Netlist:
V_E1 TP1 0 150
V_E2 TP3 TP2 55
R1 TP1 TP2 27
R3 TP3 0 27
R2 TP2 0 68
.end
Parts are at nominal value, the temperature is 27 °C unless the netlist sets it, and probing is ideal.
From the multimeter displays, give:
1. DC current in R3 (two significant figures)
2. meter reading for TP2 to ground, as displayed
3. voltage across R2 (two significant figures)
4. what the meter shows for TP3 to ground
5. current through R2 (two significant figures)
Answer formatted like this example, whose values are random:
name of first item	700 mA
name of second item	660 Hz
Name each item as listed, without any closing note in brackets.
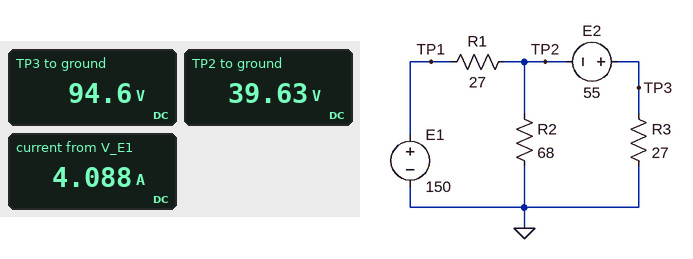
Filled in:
DC current in R3	3.5 A
meter reading for TP2 to ground, as displayed	39.63 V
voltage across R2	40 V
what the meter shows for TP3 to ground	94.6 V
current through R2	580 mA
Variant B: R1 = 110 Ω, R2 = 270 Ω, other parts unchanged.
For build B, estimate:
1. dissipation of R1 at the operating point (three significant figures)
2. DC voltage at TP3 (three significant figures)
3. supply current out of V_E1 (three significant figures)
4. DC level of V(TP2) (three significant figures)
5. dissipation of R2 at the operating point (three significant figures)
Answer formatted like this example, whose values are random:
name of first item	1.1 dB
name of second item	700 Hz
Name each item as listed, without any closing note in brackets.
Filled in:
dissipation of R1 at the operating point	243 W
DC voltage at TP3	41.5 V
supply current out of V_E1	1.49 A
DC level of V(TP2)	-13.5 V
dissipation of R2 at the operating point	676 mW
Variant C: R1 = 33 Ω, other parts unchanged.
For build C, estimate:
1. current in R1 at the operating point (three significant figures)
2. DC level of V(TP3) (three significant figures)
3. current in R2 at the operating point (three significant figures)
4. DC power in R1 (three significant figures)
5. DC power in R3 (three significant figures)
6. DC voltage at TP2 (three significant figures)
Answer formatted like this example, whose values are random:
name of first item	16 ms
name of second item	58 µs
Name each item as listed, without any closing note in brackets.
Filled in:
current in R1 at the operating point	3.62 A
DC level of V(TP3)	85.6 V
current in R2 at the operating point	450 mA
DC power in R1	432 W
DC power in R3	271 W
DC voltage at TP2	30.6 V
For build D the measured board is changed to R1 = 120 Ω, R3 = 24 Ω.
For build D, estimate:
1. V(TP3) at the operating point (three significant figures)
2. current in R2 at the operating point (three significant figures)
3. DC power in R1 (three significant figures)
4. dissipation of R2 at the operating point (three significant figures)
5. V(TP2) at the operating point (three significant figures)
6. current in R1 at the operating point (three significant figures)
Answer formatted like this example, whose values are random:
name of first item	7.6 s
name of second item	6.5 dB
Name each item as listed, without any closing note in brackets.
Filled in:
V(TP3) at the operating point	38.9 V
current in R2 at the operating point	237 mA
DC power in R1	230 W
dissipation of R2 at the operating point	3.81 W
V(TP2) at the operating point	-16.1 V
current in R1 at the operating point	1.38 A
